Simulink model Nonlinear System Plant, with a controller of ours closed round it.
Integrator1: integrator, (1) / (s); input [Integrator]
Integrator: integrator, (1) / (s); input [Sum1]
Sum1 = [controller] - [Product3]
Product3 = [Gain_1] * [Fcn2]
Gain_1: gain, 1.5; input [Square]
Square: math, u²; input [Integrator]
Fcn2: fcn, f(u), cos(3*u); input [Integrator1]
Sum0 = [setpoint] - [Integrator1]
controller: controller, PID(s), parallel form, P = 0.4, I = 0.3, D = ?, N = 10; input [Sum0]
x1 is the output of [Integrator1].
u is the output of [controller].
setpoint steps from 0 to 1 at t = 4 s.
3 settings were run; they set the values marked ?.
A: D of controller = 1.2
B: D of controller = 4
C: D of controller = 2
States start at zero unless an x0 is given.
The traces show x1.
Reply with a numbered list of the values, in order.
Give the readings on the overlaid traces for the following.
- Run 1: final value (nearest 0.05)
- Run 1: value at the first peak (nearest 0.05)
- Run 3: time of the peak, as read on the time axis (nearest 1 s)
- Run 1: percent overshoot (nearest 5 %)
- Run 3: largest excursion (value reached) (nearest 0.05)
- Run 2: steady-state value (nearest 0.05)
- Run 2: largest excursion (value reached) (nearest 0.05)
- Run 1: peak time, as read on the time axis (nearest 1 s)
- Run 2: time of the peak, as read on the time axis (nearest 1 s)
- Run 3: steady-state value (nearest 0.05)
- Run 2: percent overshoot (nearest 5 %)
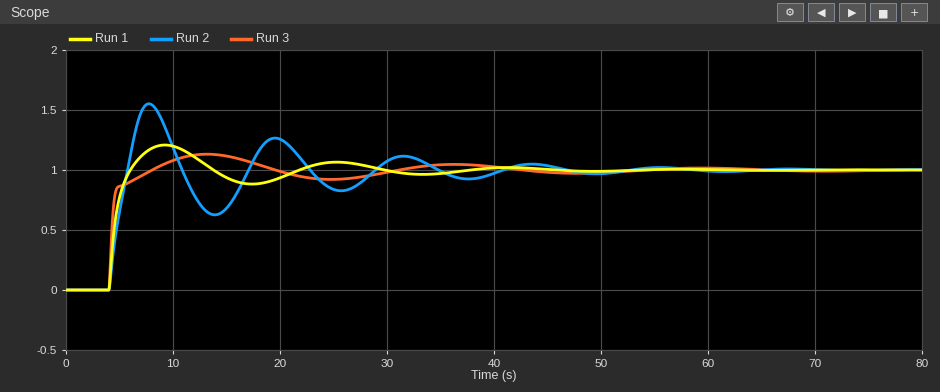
1. 1.00
2. 1.20
3. 13 s
4. 20 %
5. 1.15
6. 1.00
7. 1.55
8. 9 s
9. 8 s
10. 1.00
11. 55 %
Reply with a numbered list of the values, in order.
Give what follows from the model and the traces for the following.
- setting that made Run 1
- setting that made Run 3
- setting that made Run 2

1. C
2. B
3. A
